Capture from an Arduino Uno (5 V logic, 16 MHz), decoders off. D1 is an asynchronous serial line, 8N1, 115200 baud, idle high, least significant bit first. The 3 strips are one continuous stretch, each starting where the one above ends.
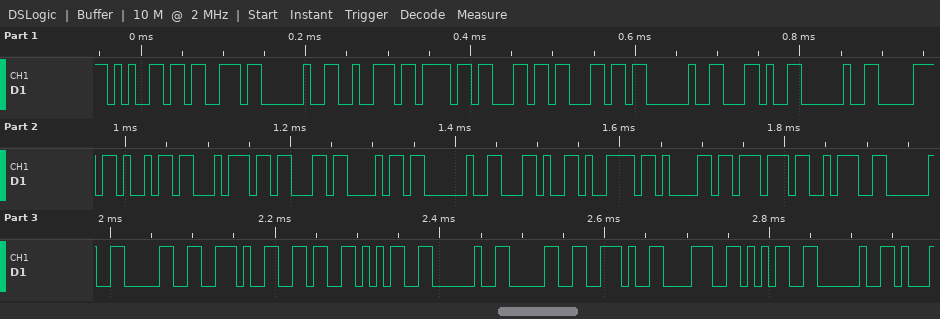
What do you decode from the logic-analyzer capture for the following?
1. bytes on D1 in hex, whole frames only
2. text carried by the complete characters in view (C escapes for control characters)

65 73 20 72 6F 6C 6C 20 2C 20 70 69 74 63 68 20 2C 79 61 77 3A 20 30 2E 36 35 20 30 2E 38 35 20
"es roll , pitch ,yaw: 0.65 0.85 "
